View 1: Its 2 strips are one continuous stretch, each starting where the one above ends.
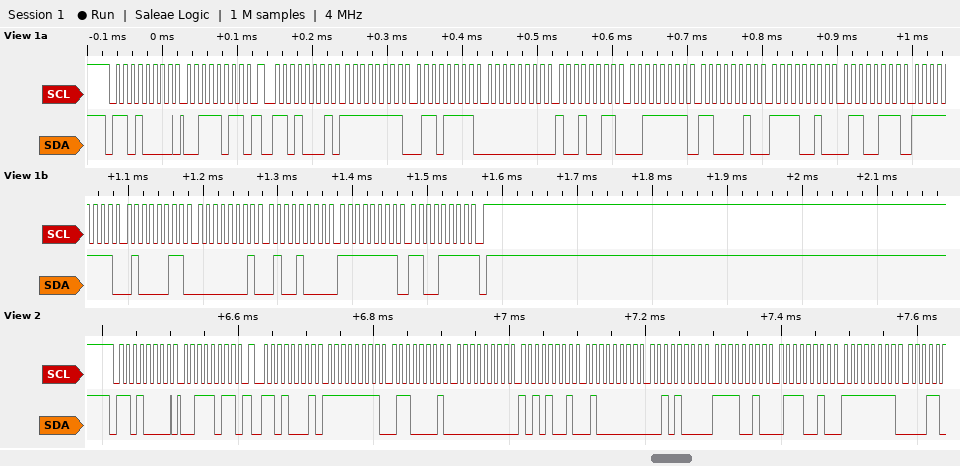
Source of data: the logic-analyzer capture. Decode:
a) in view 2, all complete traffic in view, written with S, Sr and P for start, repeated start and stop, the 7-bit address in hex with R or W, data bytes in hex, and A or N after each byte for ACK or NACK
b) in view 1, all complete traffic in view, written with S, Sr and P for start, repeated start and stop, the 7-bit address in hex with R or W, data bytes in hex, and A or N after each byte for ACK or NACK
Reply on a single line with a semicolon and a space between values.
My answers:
S 68W A 3B A Sr 68R A FF A 61 A 00 A A9 A 40 A 28 A F2 A 72 A FF A; S 68W A 3B A Sr 68R A FF A 6F A 00 A 93 A 3F A C2 A F2 A 67 A FF A 43 A 01 A 48 A FF A CF N P
